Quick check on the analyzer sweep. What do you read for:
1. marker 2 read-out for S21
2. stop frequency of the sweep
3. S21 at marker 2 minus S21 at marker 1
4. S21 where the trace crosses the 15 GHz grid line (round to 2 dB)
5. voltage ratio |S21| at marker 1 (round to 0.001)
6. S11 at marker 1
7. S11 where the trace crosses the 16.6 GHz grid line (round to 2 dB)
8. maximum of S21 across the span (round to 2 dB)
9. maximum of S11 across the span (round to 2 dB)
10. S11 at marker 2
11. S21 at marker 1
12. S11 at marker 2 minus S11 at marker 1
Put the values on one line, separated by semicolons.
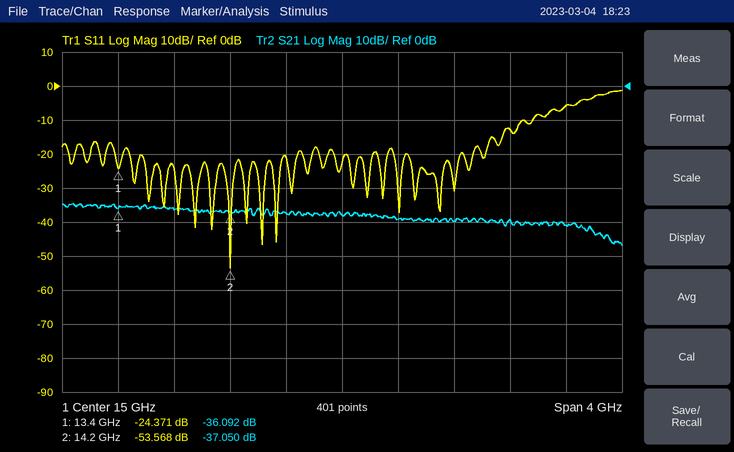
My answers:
-37.050 dB; 17 GHz; -0.958 dB; -38 dB; 0.016; -24.371 dB; -6 dB; -34 dB; -2 dB; -53.568 dB; -36.092 dB; -29.197 dB
